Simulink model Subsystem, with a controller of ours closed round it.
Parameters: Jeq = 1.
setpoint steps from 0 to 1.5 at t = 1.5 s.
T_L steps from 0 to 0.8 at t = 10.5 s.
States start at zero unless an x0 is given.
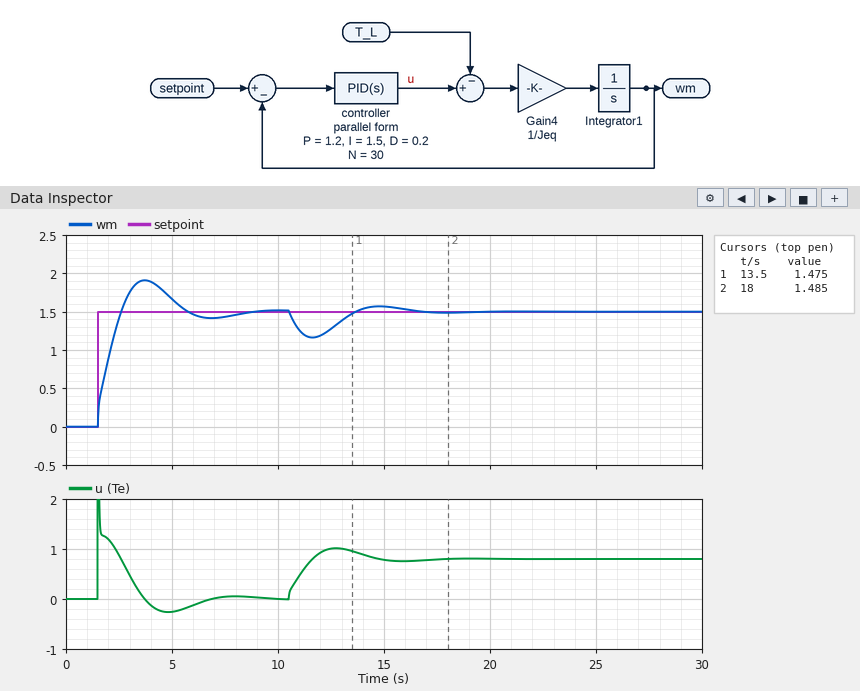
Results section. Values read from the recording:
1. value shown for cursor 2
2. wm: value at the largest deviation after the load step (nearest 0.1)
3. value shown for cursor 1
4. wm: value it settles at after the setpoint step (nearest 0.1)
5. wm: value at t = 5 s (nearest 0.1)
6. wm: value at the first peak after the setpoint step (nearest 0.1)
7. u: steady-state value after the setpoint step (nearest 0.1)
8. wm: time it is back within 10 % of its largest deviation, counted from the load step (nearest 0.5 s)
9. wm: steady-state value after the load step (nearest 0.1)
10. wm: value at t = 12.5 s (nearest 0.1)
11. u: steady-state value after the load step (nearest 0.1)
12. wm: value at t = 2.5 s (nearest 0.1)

1.485
1.2
1.475
1.5
1.7
1.9
0.0
5.5 s
1.5
1.3
0.8
1.4
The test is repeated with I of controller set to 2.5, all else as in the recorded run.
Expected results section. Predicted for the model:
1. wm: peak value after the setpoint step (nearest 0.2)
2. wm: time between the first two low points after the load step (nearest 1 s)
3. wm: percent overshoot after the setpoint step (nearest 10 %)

2.0
5 s
30 %
